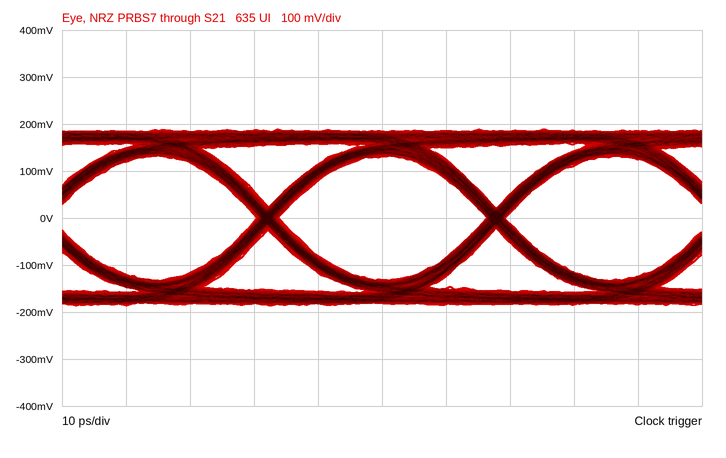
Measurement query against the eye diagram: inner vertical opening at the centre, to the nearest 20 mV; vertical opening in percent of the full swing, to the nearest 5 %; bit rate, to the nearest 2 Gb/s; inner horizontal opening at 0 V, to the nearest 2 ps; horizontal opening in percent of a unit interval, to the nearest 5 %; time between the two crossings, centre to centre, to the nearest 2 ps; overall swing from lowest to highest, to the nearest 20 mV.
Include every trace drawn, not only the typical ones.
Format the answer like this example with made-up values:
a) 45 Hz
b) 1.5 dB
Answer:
a) 260 mV
b) 70 %
c) 28 Gb/s
d) 32 ps
e) 90 %
f) 36 ps
g) 380 mV
